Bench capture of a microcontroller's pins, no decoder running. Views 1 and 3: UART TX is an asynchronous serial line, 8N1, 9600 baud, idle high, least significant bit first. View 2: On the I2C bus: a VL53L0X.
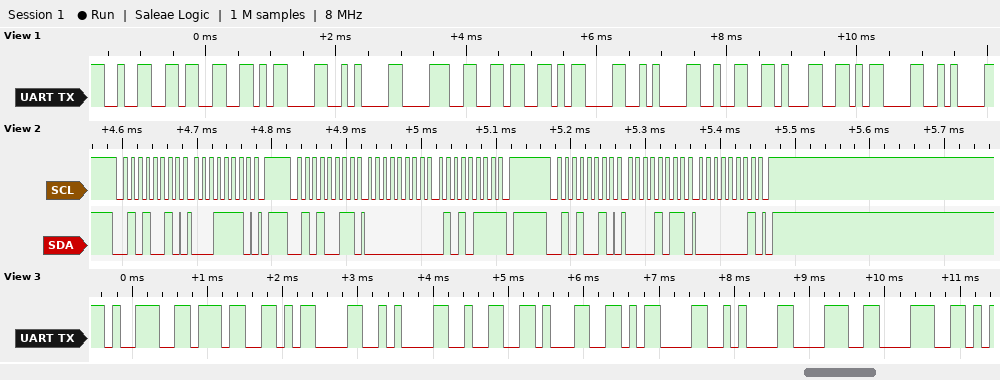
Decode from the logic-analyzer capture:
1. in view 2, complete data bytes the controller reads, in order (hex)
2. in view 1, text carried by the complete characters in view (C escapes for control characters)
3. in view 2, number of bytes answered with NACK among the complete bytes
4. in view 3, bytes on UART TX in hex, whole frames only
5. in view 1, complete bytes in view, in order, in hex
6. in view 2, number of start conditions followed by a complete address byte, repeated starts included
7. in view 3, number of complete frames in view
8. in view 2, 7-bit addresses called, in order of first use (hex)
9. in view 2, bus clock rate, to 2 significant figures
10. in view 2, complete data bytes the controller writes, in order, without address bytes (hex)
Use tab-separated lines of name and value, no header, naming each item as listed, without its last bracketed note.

in view 2, complete data bytes the controller reads, in order	00 57
in view 1, text carried by the complete characters in view	"23\r\n86\r\n21\r\n"
in view 2, number of bytes answered with NACK among the complete bytes	1
in view 3, bytes on UART TX in hex, whole frames only	39 37 0D 0A 32 31 0D 0A 38 38
in view 1, complete bytes in view, in order, in hex	32 33 0D 0A 38 36 0D 0A 32 31 0D 0A
in view 2, number of start conditions followed by a complete address byte, repeated starts included	3
in view 3, number of complete frames in view	10
in view 2, 7-bit addresses called, in order of first use	0x29
in view 2, bus clock rate, to 2 significant figures	100 kHz
in view 2, complete data bytes the controller writes, in order, without address bytes	1E 0B 01
